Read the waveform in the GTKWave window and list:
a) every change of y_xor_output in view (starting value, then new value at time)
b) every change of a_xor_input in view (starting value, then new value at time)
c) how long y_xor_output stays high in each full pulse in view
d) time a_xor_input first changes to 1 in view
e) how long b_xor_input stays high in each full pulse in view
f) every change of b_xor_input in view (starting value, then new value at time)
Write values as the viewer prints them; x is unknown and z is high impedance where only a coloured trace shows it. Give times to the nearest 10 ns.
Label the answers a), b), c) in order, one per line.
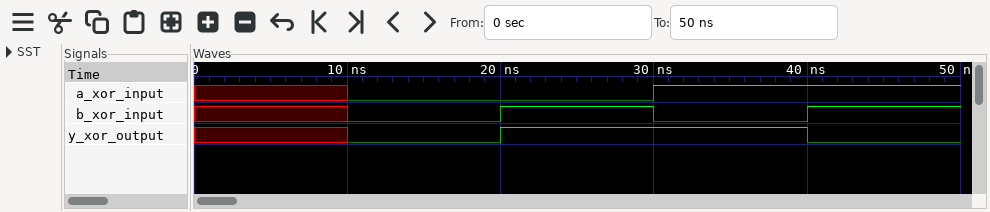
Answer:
a) x, 0 at 10 ns, 1 at 20 ns, 0 at 40 ns
b) x, 0 at 10 ns, 1 at 30 ns
c) 20 ns
d) 30 ns
e) 10 ns
f) x, 0 at 10 ns, 1 at 20 ns, 0 at 30 ns, 1 at 40 ns
